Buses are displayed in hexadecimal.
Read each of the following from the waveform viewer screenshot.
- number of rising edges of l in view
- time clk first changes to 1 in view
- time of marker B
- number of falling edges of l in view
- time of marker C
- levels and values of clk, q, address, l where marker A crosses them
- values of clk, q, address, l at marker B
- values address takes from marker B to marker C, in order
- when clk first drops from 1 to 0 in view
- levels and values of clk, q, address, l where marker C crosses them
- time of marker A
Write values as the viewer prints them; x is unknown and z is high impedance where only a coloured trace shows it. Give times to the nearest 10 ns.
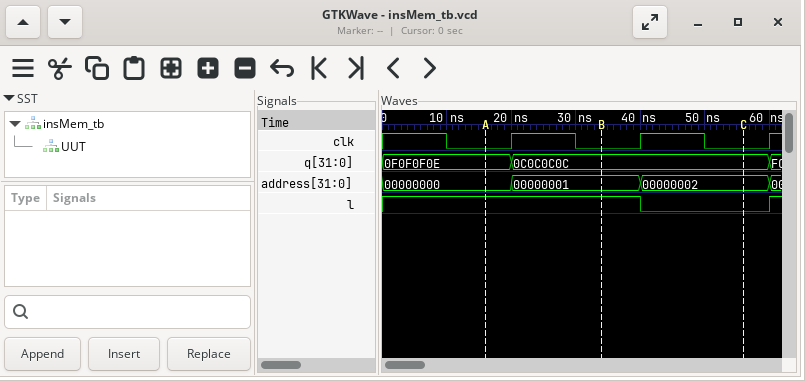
1
20 ns
30 ns
1
60 ns
clk=0, q=0F0F0F0E, address=00000000, l=1
clk=0, q=0C0C0C0C, address=00000001, l=1
00000001, 00000002
10 ns
clk=0, q=0C0C0C0C, address=00000002, l=0
20 ns
